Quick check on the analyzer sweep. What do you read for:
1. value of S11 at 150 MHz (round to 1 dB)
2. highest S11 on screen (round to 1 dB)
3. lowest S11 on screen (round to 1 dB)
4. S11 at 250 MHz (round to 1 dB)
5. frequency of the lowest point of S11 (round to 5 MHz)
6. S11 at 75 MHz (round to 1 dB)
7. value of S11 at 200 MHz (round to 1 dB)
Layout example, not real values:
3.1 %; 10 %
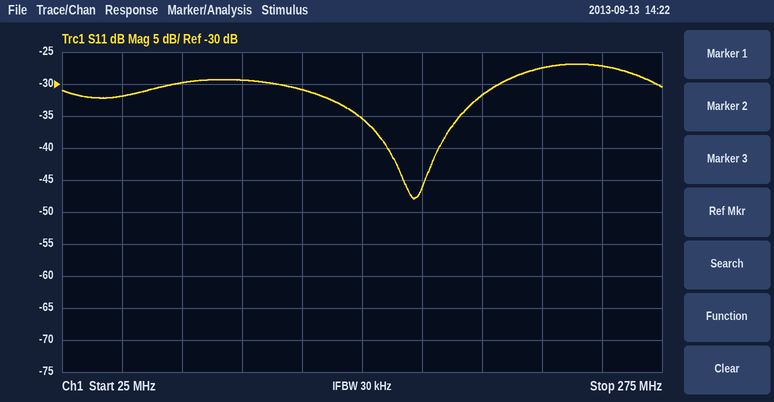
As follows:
-35 dB; -27 dB; -48 dB; -27 dB; 170 MHz; -30 dB; -32 dB
